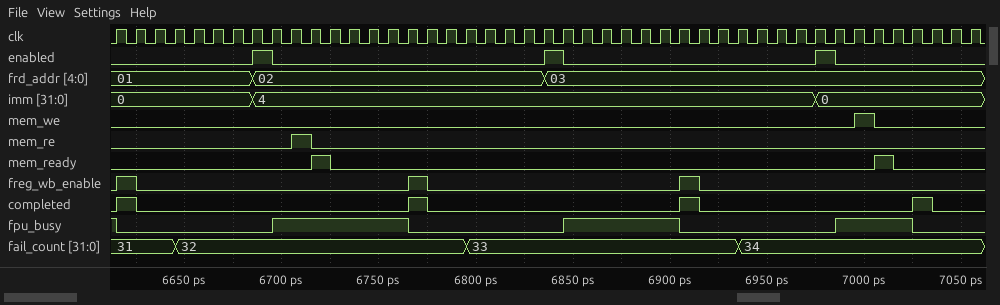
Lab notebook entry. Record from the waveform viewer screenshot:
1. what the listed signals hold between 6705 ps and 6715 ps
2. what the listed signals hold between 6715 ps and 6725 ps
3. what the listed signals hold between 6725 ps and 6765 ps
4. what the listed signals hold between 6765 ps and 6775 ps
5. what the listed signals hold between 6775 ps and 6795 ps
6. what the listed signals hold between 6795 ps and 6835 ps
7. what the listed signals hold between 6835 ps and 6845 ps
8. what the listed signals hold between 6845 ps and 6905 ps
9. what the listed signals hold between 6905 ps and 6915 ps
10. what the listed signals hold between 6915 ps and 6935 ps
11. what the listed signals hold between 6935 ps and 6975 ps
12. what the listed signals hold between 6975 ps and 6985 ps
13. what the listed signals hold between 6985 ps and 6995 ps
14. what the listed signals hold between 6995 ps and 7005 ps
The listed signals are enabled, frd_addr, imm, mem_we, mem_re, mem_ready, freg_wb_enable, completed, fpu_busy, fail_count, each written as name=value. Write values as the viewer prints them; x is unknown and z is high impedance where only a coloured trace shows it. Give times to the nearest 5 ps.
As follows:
enabled=0, frd_addr=02, imm=4, mem_we=0, mem_re=1, mem_ready=0, freg_wb_enable=0, completed=0, fpu_busy=1, fail_count=32
enabled=0, frd_addr=02, imm=4, mem_we=0, mem_re=0, mem_ready=1, freg_wb_enable=0, completed=0, fpu_busy=1, fail_count=32
enabled=0, frd_addr=02, imm=4, mem_we=0, mem_re=0, mem_ready=0, freg_wb_enable=0, completed=0, fpu_busy=1, fail_count=32
enabled=0, frd_addr=02, imm=4, mem_we=0, mem_re=0, mem_ready=0, freg_wb_enable=1, completed=1, fpu_busy=0, fail_count=32
enabled=0, frd_addr=02, imm=4, mem_we=0, mem_re=0, mem_ready=0, freg_wb_enable=0, completed=0, fpu_busy=0, fail_count=32
enabled=0, frd_addr=02, imm=4, mem_we=0, mem_re=0, mem_ready=0, freg_wb_enable=0, completed=0, fpu_busy=0, fail_count=33
enabled=1, frd_addr=03, imm=4, mem_we=0, mem_re=0, mem_ready=0, freg_wb_enable=0, completed=0, fpu_busy=0, fail_count=33
enabled=0, frd_addr=03, imm=4, mem_we=0, mem_re=0, mem_ready=0, freg_wb_enable=0, completed=0, fpu_busy=1, fail_count=33
enabled=0, frd_addr=03, imm=4, mem_we=0, mem_re=0, mem_ready=0, freg_wb_enable=1, completed=1, fpu_busy=0, fail_count=33
enabled=0, frd_addr=03, imm=4, mem_we=0, mem_re=0, mem_ready=0, freg_wb_enable=0, completed=0, fpu_busy=0, fail_count=33
enabled=0, frd_addr=03, imm=4, mem_we=0, mem_re=0, mem_ready=0, freg_wb_enable=0, completed=0, fpu_busy=0, fail_count=34
enabled=1, frd_addr=03, imm=0, mem_we=0, mem_re=0, mem_ready=0, freg_wb_enable=0, completed=0, fpu_busy=0, fail_count=34
enabled=0, frd_addr=03, imm=0, mem_we=0, mem_re=0, mem_ready=0, freg_wb_enable=0, completed=0, fpu_busy=1, fail_count=34
enabled=0, frd_addr=03, imm=0, mem_we=1, mem_re=0, mem_ready=0, freg_wb_enable=0, completed=0, fpu_busy=1, fail_count=34
